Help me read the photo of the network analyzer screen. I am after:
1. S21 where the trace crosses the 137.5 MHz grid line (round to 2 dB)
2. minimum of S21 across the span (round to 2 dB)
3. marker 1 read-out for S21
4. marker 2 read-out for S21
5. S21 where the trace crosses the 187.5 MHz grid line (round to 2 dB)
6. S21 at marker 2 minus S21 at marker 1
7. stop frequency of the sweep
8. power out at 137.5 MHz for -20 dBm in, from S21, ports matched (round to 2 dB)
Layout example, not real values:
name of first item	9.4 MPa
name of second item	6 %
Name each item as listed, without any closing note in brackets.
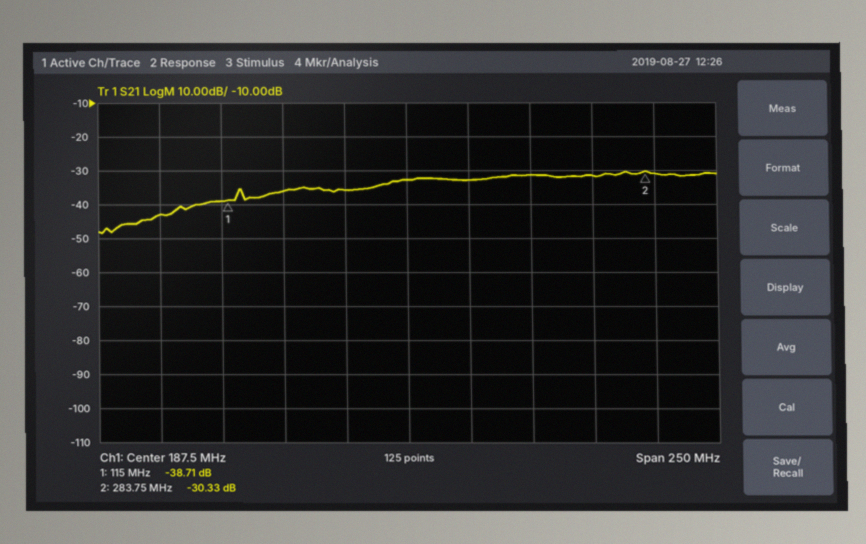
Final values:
S21 where the trace crosses the 137.5 MHz grid line	-36 dB
minimum of S21 across the span	-48 dB
marker 1 read-out for S21	-38.71 dB
marker 2 read-out for S21	-30.33 dB
S21 where the trace crosses the 187.5 MHz grid line	-32 dB
S21 at marker 2 minus S21 at marker 1	8.38 dB
stop frequency of the sweep	312.5 MHz
power out at 137.5 MHz for -20 dBm in, from S21, ports matched	-56 dBm
